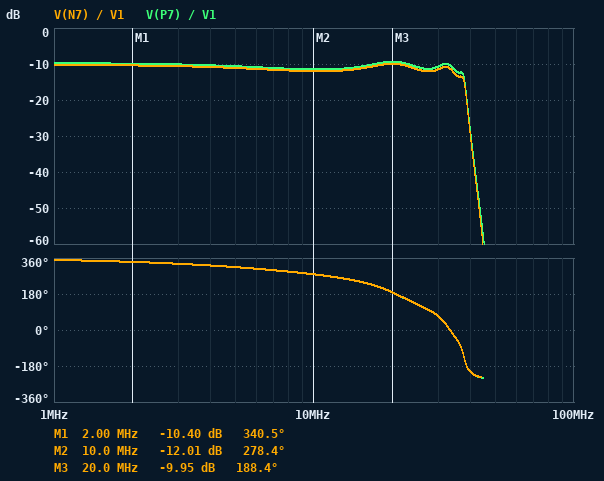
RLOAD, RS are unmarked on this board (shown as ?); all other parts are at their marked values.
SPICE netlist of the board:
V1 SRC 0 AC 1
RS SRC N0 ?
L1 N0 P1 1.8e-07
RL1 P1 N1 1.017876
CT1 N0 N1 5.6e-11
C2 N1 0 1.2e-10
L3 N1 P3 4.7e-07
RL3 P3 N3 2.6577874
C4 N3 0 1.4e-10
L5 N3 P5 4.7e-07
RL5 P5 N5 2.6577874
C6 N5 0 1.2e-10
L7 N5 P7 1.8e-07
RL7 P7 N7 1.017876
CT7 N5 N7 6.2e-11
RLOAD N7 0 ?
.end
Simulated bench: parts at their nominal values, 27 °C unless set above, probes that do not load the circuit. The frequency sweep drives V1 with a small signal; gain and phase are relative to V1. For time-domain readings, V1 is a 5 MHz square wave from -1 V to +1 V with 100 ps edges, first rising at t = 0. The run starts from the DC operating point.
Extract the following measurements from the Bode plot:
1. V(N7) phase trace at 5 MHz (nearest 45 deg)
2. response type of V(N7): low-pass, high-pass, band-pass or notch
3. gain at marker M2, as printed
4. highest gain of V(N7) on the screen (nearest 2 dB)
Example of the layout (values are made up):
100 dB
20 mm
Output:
315 deg
low-pass
-12.01 dB
-10 dB
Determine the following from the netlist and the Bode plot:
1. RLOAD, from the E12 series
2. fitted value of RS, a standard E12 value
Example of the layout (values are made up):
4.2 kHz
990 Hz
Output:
18 Ω
33 Ω
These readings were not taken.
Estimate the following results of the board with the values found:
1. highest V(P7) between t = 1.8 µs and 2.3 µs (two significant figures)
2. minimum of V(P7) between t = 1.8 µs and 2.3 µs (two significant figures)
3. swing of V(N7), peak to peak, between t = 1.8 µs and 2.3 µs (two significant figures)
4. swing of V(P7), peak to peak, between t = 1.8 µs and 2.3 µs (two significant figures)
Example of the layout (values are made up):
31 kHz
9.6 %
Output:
390 mV
-390 mV
730 mV
780 mV
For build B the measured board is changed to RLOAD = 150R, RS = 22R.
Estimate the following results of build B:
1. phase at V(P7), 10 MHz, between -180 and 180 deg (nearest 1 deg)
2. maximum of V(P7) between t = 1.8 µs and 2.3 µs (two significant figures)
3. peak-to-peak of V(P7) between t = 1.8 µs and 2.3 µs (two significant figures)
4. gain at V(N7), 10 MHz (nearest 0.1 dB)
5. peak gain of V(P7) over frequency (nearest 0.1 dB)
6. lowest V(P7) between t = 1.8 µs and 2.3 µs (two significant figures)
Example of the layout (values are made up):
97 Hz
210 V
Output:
-78 deg
1.5 V
3.0 V
1.4 dB
1.5 dB
-1.5 V
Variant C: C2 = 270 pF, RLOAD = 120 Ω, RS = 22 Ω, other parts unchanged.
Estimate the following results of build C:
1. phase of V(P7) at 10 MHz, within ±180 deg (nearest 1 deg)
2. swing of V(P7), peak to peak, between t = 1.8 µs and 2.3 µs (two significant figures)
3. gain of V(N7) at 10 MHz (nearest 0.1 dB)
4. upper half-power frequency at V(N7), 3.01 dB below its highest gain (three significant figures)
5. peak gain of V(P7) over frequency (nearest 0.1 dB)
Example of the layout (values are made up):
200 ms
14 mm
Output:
-88 deg
2.9 V
0.4 dB
25.6 MHz
0.6 dB
